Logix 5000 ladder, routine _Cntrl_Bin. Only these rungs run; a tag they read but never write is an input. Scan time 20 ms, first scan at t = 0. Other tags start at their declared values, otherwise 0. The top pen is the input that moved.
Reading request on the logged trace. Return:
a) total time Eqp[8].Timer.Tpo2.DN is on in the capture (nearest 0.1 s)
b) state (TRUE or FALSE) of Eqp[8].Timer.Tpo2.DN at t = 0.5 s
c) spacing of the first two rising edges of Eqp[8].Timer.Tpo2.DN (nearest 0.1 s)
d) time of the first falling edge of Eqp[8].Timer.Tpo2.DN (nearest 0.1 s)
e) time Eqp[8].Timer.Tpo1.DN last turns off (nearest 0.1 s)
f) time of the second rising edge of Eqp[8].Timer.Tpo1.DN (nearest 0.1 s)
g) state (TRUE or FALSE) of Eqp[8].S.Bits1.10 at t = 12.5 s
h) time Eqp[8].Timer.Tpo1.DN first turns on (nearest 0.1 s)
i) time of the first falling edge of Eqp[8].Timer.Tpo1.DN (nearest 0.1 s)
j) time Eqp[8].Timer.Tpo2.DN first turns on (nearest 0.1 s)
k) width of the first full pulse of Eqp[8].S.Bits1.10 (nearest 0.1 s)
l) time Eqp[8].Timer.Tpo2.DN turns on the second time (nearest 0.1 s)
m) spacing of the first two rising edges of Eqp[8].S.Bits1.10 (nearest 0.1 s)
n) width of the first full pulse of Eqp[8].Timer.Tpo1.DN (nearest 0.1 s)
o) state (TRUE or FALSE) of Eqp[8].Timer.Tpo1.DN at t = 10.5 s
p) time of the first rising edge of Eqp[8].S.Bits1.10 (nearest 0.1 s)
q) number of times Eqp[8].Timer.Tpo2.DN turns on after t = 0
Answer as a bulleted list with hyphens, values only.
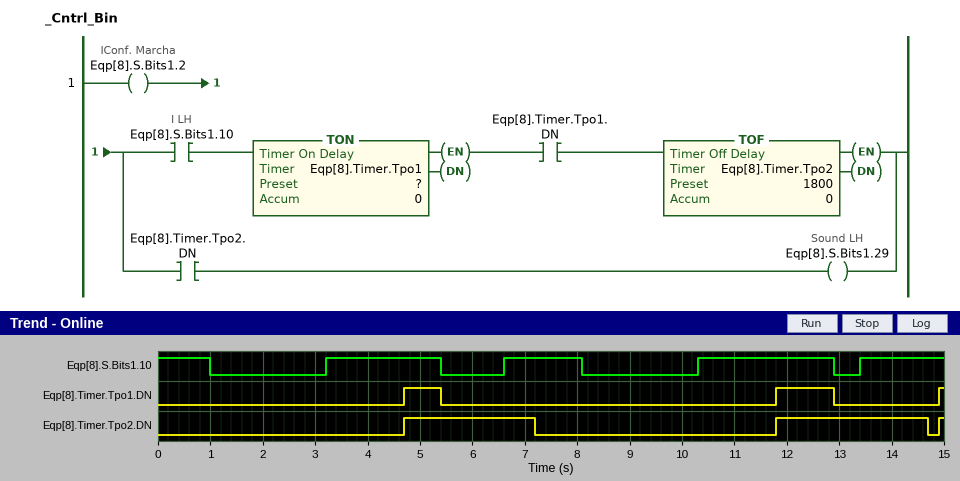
- 5.5 s
- FALSE
- 7.1 s
- 7.2 s
- 12.9 s
- 11.8 s
- TRUE
- 4.7 s
- 5.4 s
- 4.7 s
- 2.2 s
- 11.8 s
- 3.4 s
- 0.7 s
- FALSE
- 3.2 s
- 3
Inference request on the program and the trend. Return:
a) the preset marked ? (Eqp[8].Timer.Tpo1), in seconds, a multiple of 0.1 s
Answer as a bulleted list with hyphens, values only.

- 1.5 s
